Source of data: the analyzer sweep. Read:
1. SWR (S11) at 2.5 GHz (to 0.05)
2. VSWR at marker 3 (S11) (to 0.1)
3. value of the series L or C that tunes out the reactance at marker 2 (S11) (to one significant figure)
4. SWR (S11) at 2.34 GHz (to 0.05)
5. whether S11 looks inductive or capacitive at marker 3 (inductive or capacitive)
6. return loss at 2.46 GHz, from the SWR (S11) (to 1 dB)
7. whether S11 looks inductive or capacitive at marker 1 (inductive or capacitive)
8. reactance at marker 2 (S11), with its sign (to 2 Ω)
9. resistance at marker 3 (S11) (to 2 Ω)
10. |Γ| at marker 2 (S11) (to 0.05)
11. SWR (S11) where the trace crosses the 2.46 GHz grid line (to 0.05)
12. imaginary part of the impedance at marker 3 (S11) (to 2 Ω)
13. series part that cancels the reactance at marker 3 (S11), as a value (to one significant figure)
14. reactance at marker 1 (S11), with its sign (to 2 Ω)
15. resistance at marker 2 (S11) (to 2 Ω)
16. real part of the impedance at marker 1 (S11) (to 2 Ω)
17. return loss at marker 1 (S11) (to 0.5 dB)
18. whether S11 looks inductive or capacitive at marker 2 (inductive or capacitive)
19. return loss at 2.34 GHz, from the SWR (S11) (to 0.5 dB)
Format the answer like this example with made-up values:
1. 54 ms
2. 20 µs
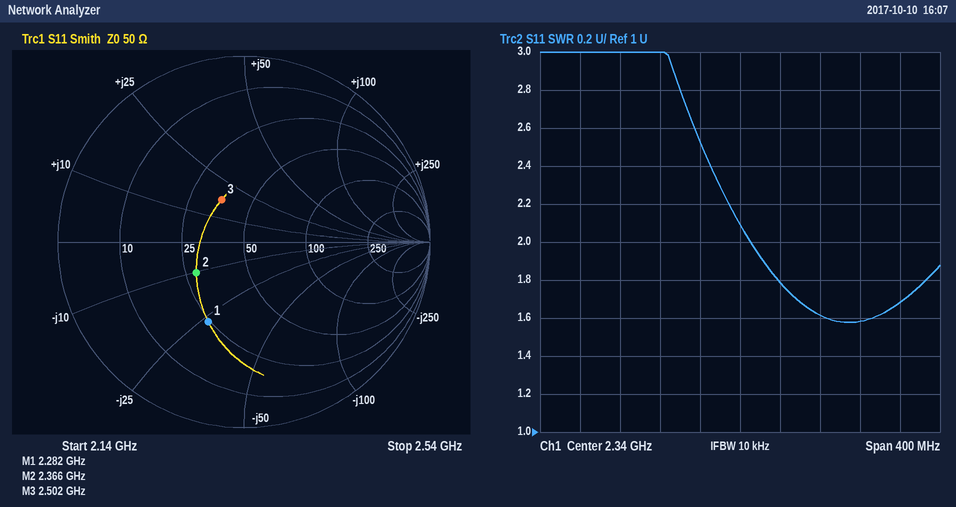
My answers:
1. 1.70
2. 1.7
3. 700 pH
4. 2.10
5. inductive
6. 13 dB
7. capacitive
8. -10 Ω
9. 36 Ω
10. 0.30
11. 1.60
12. +18 Ω
13. 4 pF
14. -26 Ω
15. 28 Ω
16. 24 Ω
17. 6.5 dB
18. capacitive
19. 9.0 dB
